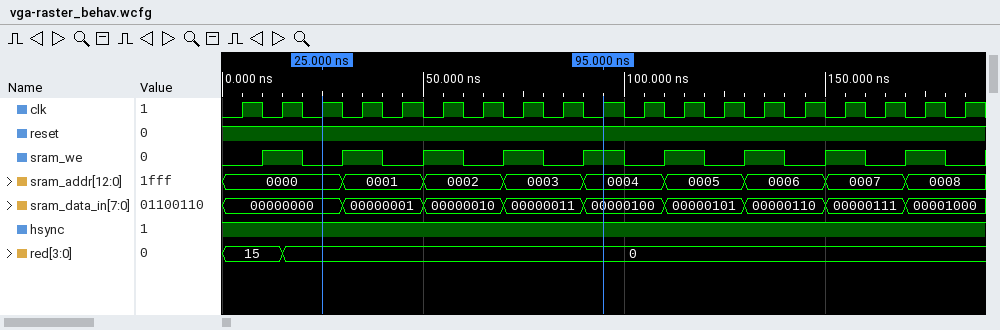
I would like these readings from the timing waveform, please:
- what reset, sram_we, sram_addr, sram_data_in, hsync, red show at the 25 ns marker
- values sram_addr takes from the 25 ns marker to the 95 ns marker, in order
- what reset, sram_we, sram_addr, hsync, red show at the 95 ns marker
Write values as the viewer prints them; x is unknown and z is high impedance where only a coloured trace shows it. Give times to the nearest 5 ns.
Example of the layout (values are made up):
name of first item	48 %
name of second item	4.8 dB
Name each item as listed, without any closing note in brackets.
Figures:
what reset, sram_we, sram_addr, sram_data_in, hsync, red show at the 25 ns marker	reset=1, sram_we=0, sram_addr=0000, sram_data_in=00000000, hsync=1, red=0
values sram_addr takes from the 25 ns marker to the 95 ns marker, in order	0000, 0001, 0002, 0003, 0004
what reset, sram_we, sram_addr, hsync, red show at the 95 ns marker	reset=1, sram_we=1, sram_addr=0004, hsync=1, red=0
